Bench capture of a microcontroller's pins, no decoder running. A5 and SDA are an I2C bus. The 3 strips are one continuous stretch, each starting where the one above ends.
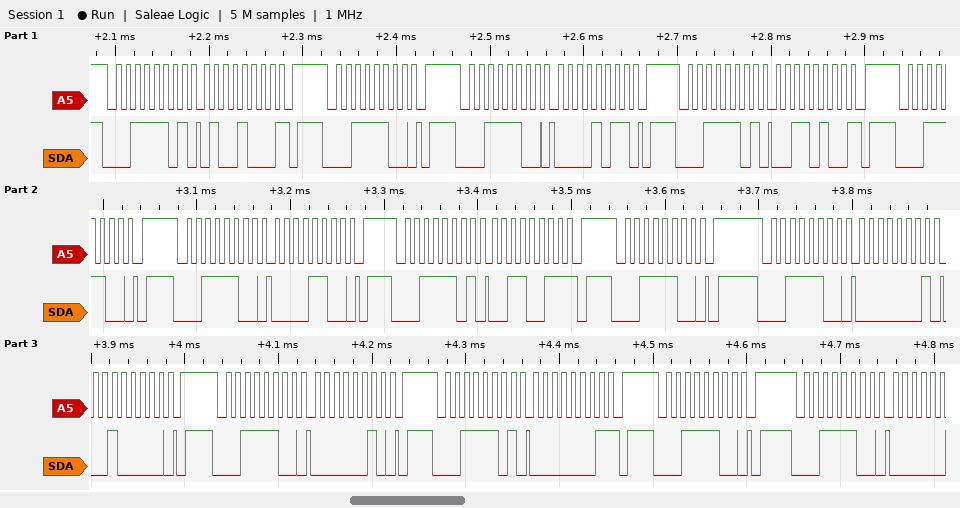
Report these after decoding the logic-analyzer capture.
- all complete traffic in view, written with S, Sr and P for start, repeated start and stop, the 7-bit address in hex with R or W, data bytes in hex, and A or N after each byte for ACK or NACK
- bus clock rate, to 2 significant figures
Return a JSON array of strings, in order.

["S 1ER A 48 N P S 1EW A P S 1EW A 0B A P S 1ER A 34 N P S 1EW A P S 1EW A 0C A P S 1ER A 33 N P S 1EW A P S 1EW A 01 A 20 A P S 1EW A 02 A P S 1ER A 01 N P S 1EW A P S 1EW A", "100 kHz"]
